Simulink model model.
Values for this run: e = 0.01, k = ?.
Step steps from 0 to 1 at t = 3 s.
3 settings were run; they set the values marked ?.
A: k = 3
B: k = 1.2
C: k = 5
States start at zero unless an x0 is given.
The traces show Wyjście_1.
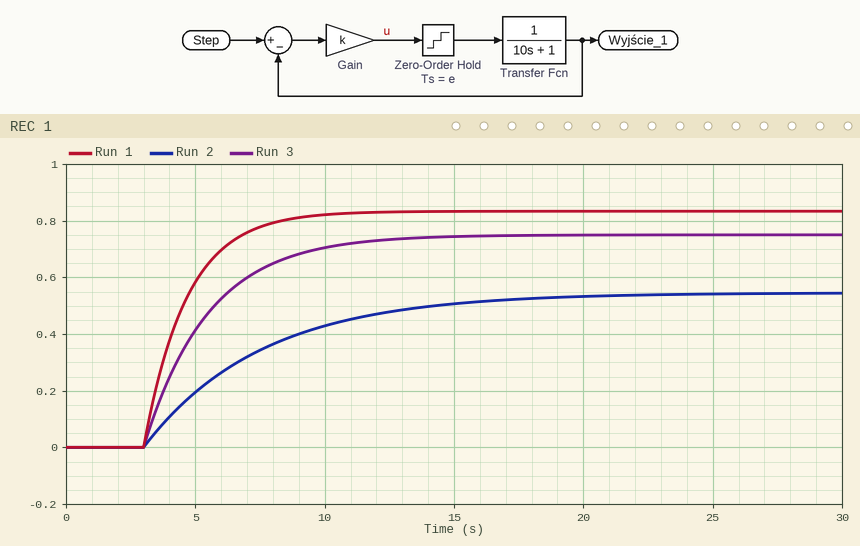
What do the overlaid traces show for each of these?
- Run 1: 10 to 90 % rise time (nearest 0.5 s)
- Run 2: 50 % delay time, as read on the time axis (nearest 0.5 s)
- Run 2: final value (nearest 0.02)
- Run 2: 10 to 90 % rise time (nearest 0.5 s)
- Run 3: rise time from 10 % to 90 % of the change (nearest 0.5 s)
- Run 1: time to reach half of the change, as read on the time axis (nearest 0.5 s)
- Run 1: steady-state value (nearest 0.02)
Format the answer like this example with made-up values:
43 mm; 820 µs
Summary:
3.5 s; 6.0 s; 0.54; 10.0 s; 5.5 s; 4.0 s; 0.84
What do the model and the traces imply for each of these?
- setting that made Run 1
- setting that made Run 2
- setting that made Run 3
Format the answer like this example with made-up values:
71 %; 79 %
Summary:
C; B; A
